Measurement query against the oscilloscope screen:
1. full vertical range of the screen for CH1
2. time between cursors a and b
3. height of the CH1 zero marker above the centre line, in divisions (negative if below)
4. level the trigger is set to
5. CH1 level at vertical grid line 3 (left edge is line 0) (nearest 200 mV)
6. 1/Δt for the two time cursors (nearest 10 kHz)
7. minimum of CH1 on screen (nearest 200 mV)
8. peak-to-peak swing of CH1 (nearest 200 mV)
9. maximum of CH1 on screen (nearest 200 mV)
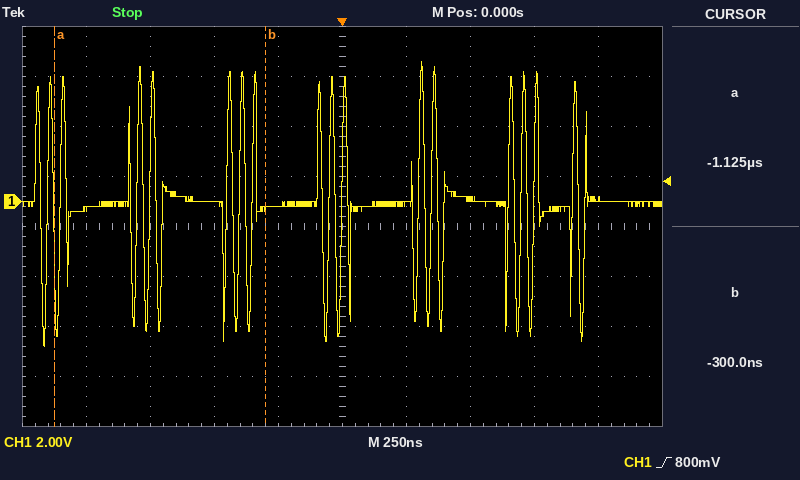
16 V
825 ns
+0.5 div
800 mV
0.0 V
1.21 MHz
-5.8 V
11.4 V
5.6 V
